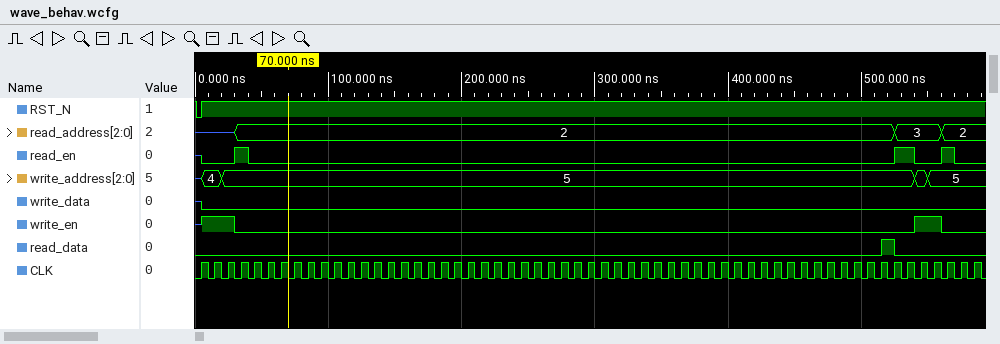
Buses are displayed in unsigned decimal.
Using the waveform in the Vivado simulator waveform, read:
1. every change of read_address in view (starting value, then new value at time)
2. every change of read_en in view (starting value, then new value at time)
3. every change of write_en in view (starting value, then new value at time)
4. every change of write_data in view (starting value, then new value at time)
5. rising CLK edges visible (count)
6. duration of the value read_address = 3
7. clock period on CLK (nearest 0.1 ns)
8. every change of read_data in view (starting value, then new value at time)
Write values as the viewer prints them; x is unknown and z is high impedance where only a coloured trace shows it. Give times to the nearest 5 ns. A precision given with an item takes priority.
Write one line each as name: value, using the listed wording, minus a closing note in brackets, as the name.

every change of read_address in view: z, 2 at 30 ns, 3 at 525 ns, 2 at 560 ns
every change of read_en in view: z, 0 at 5 ns, 1 at 30 ns, 0 at 40 ns, 1 at 525 ns, 0 at 540 ns, 1 at 560 ns, 0 at 570 ns
every change of write_en in view: z, 1 at 5 ns, 0 at 30 ns, 1 at 540 ns, 0 at 560 ns
every change of write_data in view: z, 0 at 5 ns
rising CLK edges visible: 59
duration of the value read_address = 3: 35 ns
clock period on CLK: 10 ns
every change of read_data in view: 0, 1 at 515 ns, 0 at 525 ns
